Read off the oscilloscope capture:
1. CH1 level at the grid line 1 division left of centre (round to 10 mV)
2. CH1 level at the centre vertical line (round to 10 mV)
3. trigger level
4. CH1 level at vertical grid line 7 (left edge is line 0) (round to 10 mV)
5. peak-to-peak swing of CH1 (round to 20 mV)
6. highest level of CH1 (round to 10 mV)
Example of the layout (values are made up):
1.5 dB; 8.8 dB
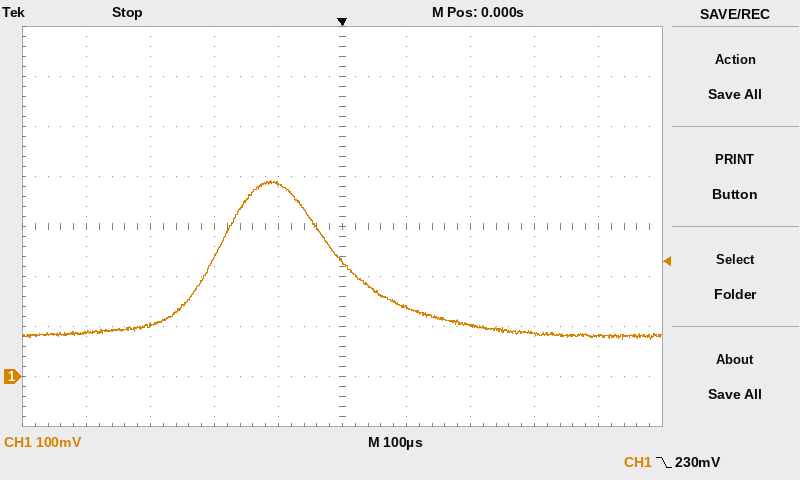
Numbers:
390 mV; 230 mV; 230 mV; 100 mV; 320 mV; 390 mV
